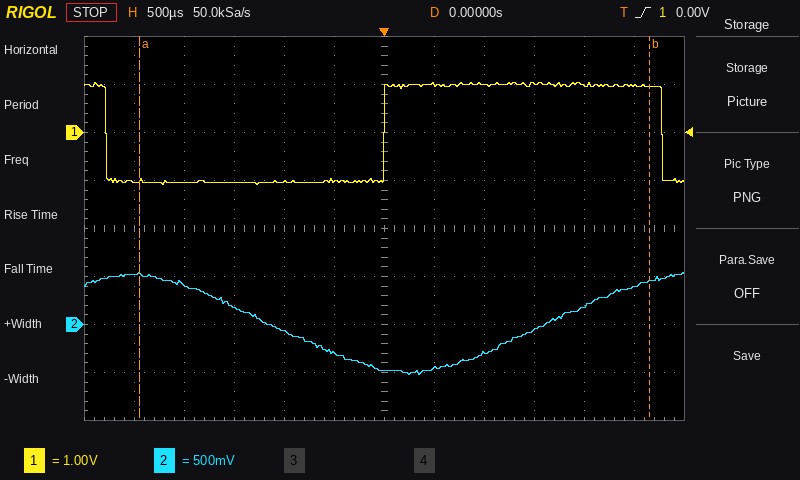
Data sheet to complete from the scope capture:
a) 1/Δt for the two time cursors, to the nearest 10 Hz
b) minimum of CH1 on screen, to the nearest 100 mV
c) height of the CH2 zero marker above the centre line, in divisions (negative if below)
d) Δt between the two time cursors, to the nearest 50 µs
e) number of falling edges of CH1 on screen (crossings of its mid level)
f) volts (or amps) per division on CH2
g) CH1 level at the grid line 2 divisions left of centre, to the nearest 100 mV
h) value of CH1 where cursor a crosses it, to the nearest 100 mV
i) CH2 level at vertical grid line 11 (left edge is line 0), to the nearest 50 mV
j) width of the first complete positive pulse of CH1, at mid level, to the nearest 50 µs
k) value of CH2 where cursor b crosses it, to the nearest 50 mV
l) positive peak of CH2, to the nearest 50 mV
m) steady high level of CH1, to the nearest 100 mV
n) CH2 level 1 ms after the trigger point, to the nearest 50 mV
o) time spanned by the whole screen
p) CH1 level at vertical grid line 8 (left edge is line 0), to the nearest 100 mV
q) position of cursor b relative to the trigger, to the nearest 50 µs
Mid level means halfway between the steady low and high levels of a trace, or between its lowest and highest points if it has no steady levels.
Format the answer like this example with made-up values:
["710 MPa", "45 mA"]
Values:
["200 Hz", "-1.1 V", "-2.0 div", "5.10 ms", "2", "500 mV", "-1.0 V", "-1.0 V", "400 mV", "2.80 ms", "450 mV", "550 mV", "1.0 V", "-300 mV", "6 ms", "1.0 V", "+2.65 ms"]
